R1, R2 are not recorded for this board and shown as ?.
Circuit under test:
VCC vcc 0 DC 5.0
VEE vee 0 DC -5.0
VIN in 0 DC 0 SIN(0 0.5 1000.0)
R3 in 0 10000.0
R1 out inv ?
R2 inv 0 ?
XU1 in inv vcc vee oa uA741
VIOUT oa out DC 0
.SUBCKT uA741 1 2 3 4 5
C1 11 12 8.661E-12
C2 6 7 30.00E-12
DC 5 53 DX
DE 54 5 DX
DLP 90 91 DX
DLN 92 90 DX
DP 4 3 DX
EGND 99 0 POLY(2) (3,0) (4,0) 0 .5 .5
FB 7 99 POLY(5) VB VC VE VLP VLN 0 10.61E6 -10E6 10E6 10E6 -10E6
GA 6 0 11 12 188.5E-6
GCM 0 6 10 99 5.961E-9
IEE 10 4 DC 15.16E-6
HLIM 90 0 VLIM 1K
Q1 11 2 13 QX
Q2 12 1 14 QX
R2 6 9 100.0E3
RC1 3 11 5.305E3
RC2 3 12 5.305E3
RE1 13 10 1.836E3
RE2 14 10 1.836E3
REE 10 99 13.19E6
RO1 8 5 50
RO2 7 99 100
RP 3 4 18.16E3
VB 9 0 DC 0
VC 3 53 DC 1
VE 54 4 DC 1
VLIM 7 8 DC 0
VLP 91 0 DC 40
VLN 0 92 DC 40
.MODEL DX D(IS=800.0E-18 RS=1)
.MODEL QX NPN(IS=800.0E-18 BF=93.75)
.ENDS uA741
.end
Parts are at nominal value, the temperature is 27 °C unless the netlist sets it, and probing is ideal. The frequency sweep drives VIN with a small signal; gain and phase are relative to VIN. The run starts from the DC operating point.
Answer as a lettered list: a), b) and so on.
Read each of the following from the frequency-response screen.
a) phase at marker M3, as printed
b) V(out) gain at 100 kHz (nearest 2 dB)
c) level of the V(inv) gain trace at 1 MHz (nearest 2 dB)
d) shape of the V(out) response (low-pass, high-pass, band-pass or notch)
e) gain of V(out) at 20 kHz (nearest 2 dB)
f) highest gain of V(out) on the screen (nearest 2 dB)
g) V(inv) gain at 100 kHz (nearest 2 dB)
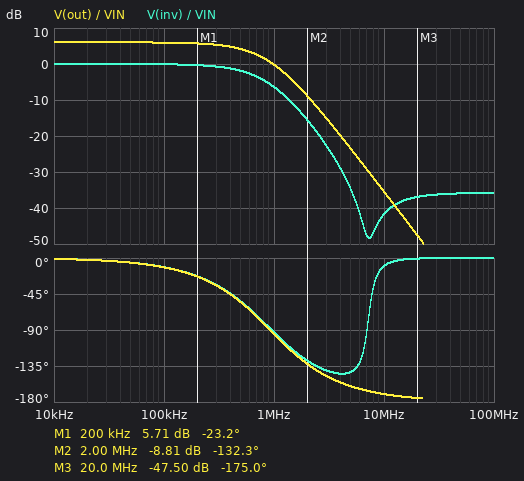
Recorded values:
a) -175.0 deg
b) 6 dB
c) -6 dB
d) low-pass
e) 6 dB
f) 6 dB
g) 0 dB
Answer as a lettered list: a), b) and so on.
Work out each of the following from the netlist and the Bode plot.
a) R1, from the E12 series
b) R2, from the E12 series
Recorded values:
a) 33 kΩ
b) 33 kΩ
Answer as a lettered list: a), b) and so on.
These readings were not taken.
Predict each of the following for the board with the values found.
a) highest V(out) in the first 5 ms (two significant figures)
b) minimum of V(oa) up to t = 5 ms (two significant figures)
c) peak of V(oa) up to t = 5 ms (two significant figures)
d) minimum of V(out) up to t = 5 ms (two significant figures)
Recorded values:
a) 1.0 V
b) -1.0 V
c) 1.0 V
d) -1.0 V
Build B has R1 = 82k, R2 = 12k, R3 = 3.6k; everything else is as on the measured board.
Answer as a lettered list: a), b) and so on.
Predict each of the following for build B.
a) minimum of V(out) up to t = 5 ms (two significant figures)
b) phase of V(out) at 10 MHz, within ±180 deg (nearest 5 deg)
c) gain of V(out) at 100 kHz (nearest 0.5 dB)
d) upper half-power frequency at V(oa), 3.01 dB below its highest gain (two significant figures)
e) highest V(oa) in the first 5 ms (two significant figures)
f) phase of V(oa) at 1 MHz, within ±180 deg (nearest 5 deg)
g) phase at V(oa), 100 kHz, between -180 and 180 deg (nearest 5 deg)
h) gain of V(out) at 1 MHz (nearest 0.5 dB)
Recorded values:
a) -3.9 V
b) -170 deg
c) 16.0 dB
d) 140 kHz
e) 3.9 V
f) -115 deg
g) -40 deg
h) -1.0 dB
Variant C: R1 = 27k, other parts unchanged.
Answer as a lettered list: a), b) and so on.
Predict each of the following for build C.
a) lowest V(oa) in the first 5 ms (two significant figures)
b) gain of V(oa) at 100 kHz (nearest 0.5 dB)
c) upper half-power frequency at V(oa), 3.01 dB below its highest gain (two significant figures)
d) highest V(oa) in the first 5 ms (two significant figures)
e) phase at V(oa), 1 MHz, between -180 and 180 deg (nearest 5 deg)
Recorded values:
a) -910 mV
b) 5.0 dB
c) 730 kHz
d) 910 mV
e) -90 deg
